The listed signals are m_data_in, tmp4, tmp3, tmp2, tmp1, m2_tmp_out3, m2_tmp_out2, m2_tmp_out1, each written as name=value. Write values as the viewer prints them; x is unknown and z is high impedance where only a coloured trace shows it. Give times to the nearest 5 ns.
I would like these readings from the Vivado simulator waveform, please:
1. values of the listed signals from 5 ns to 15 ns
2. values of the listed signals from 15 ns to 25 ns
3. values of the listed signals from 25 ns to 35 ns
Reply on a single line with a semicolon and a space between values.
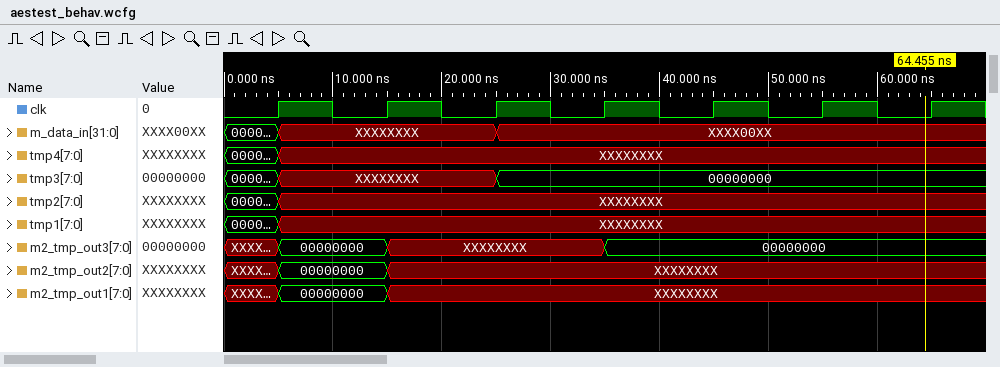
m_data_in=XXXXXXXX, tmp4=XXXXXXXX, tmp3=XXXXXXXX, tmp2=XXXXXXXX, tmp1=XXXXXXXX, m2_tmp_out3=00000000, m2_tmp_out2=00000000, m2_tmp_out1=00000000; m_data_in=XXXXXXXX, tmp4=XXXXXXXX, tmp3=XXXXXXXX, tmp2=XXXXXXXX, tmp1=XXXXXXXX, m2_tmp_out3=XXXXXXXX, m2_tmp_out2=XXXXXXXX, m2_tmp_out1=XXXXXXXX; m_data_in=XXXX00XX, tmp4=XXXXXXXX, tmp3=00000000, tmp2=XXXXXXXX, tmp1=XXXXXXXX, m2_tmp_out3=XXXXXXXX, m2_tmp_out2=XXXXXXXX, m2_tmp_out1=XXXXXXXX
